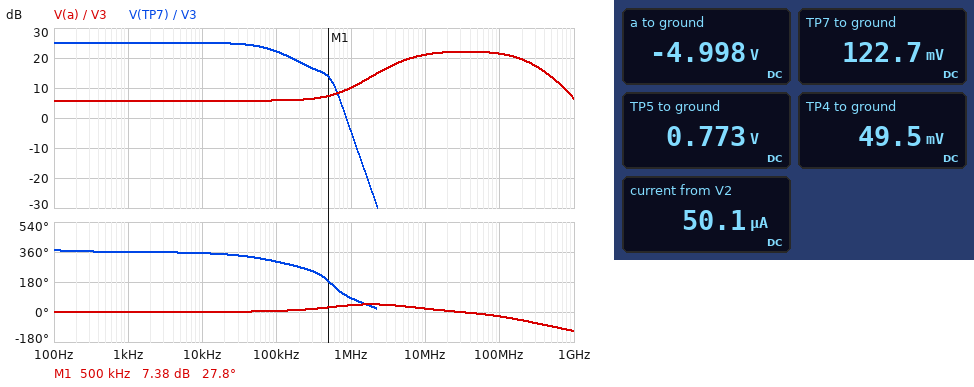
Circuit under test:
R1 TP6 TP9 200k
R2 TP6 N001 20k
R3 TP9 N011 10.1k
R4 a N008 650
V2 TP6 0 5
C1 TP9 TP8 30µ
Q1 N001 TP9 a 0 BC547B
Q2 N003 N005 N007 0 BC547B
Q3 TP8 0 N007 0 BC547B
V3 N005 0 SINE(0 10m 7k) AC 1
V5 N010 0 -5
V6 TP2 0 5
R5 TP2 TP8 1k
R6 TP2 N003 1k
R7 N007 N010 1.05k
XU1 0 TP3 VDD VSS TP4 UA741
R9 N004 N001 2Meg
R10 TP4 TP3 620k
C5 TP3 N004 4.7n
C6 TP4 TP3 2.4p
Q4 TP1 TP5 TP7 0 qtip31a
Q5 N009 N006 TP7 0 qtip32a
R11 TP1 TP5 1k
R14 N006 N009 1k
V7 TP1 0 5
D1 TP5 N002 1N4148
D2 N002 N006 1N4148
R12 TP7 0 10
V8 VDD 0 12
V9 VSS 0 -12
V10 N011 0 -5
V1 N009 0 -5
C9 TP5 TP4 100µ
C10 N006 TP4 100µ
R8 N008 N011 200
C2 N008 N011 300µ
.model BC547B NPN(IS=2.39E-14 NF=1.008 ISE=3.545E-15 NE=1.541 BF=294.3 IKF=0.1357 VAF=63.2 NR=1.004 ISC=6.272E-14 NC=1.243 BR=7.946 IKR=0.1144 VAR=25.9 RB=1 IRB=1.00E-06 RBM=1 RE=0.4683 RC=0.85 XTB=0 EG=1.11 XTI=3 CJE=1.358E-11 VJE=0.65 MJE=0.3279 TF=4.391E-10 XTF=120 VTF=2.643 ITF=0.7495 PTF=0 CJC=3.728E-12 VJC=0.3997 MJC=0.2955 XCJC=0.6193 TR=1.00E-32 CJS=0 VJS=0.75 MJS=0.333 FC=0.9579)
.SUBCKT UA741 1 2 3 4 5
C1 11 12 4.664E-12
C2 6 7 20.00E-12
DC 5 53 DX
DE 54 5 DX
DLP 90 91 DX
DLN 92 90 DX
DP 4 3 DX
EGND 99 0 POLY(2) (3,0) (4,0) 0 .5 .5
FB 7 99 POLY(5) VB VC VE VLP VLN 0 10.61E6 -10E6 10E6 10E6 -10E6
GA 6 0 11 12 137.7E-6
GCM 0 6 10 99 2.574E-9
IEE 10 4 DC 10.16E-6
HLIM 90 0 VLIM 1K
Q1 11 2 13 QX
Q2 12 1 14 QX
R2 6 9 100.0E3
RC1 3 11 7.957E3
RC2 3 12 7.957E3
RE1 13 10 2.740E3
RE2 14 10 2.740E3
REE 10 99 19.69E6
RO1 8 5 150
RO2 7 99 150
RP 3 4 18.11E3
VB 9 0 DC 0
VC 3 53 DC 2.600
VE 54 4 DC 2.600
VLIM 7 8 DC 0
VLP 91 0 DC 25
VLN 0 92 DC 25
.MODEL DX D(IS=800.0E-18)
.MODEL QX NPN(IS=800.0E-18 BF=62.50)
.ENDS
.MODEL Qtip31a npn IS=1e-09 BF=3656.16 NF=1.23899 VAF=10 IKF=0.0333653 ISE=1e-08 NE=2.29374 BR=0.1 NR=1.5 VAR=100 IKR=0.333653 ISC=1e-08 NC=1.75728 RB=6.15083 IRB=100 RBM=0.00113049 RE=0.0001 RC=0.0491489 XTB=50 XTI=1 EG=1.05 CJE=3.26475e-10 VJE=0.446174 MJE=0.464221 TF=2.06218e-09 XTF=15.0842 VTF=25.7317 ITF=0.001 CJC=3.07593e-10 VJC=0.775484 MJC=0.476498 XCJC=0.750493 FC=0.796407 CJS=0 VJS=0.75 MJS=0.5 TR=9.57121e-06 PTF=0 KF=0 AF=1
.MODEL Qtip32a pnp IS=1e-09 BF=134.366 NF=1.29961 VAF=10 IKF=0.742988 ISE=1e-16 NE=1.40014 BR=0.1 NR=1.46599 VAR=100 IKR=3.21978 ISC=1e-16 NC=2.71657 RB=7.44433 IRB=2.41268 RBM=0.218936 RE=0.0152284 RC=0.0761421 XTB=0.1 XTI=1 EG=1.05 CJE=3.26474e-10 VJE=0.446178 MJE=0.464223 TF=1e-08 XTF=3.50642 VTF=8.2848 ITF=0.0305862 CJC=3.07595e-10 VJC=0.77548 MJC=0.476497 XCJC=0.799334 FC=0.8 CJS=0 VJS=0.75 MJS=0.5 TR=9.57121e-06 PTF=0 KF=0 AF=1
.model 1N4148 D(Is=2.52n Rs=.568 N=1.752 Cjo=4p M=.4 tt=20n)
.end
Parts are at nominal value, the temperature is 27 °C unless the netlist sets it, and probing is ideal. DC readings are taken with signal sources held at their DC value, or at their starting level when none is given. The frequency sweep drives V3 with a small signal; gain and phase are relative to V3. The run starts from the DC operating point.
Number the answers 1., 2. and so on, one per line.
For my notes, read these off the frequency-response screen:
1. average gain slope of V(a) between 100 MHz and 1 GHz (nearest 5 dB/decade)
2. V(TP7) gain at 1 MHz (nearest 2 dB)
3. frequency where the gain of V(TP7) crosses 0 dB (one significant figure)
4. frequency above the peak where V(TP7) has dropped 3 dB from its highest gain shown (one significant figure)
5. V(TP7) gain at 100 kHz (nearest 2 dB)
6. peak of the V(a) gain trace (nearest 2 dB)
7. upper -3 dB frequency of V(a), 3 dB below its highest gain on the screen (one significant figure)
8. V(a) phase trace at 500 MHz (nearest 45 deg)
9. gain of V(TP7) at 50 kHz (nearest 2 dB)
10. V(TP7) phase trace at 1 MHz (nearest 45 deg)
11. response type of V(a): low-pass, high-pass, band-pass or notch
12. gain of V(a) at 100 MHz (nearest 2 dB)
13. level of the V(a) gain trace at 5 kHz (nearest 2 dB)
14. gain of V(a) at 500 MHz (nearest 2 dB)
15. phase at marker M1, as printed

1. -15 dB/decade
2. -4 dB
3. 900 kHz
4. 100 kHz
5. 22 dB
6. 22 dB
7. 200 MHz
8. -90 deg
9. 24 dB
10. 90 deg
11. band-pass
12. 22 dB
13. 6 dB
14. 14 dB
15. 27.8 deg
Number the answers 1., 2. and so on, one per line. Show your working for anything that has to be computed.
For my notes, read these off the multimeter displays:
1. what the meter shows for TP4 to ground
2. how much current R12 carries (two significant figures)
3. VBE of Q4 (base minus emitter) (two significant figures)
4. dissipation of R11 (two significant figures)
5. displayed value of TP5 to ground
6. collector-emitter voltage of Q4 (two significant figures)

1. 49.5 mV
2. (122.7 mV) / 10 Ω = 12 mA
3. 773 mV - 122.7 mV = 650 mV
4. (5 V - 773 mV)^2 / 1 kΩ = 18 mW
5. 0.773 V
6. 5 V - 122.7 mV = 4.9 V
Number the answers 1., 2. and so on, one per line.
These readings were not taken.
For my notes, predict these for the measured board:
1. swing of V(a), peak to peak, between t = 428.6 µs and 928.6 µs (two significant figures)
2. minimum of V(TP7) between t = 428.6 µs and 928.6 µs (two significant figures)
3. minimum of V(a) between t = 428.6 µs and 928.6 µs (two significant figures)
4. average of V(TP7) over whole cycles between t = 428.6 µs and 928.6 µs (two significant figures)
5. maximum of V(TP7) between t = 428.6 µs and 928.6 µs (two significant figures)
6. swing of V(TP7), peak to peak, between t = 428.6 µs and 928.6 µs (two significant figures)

1. 200 mV
2. 60 mV
3. -5.0 V
4. 570 mV
5. 1.9 V
6. 1.8 V
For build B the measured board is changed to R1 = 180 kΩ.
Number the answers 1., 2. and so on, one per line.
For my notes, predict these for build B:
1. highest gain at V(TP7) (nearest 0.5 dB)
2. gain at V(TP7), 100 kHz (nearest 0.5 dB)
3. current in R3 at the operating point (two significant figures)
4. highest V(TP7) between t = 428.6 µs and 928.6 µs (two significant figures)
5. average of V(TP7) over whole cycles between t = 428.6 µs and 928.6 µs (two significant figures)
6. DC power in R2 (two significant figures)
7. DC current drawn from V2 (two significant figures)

1. 37.0 dB
2. 34.0 dB
3. 53 µA
4. 2.2 V
5. 670 mV
6. 3.1 µW
7. 65 µA
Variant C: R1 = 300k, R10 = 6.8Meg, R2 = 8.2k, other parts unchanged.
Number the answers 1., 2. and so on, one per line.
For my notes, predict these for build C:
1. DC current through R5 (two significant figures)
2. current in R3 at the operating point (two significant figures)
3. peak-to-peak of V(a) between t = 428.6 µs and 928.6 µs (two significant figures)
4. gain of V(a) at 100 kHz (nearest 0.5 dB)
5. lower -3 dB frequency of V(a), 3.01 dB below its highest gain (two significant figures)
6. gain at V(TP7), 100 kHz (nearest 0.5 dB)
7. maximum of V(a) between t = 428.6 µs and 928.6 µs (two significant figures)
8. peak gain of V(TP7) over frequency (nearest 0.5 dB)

1. 2.1 mA
2. 32 µA
3. 73 mV
4. -13.0 dB
5. 5.3 MHz
6. -22.5 dB
7. -4.9 V
8. -12.0 dB
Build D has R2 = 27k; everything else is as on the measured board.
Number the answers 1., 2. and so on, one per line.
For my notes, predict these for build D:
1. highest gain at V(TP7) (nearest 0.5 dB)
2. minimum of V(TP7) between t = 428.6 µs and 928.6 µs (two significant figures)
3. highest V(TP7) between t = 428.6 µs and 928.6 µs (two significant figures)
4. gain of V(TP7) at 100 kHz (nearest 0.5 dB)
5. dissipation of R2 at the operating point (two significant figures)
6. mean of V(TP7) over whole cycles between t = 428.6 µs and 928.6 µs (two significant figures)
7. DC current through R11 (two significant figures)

1. 27.5 dB
2. 38 mV
3. 2.5 V
4. 24.5 dB
5. 170 nW
6. 730 mV
7. 4.2 mA
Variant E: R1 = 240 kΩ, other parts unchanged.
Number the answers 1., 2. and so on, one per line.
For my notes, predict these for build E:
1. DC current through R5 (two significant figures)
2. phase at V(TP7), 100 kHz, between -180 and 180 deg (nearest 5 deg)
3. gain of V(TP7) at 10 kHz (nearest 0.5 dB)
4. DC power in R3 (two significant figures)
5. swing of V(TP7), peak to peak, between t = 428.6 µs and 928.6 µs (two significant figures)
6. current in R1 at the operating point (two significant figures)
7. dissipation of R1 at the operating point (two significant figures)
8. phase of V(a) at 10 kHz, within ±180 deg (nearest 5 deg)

1. 2.1 mA
2. -65 deg
3. 0.5 dB
4. 16 µW
5. 1.2 V
6. 40 µA
7. 380 µW
8. 10 deg
